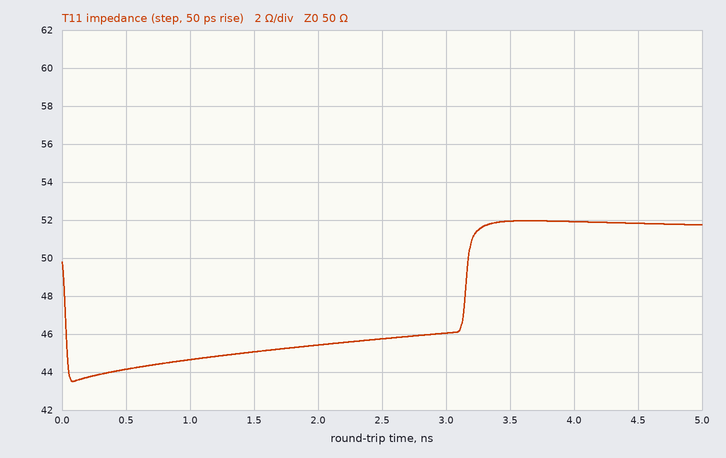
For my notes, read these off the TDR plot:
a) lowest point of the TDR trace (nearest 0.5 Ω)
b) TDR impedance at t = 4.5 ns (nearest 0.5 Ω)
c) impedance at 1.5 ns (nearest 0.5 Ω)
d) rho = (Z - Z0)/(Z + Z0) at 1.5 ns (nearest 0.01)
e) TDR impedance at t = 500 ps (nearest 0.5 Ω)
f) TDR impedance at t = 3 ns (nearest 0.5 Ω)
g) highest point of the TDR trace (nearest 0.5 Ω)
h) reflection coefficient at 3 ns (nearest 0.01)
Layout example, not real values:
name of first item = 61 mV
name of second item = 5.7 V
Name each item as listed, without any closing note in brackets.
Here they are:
lowest point of the TDR trace = 43.5 Ω
TDR impedance at t = 4.5 ns = 52.0 Ω
impedance at 1.5 ns = 45.0 Ω
rho = (Z - Z0)/(Z + Z0) at 1.5 ns = -0.05
TDR impedance at t = 500 ps = 44.0 Ω
TDR impedance at t = 3 ns = 46.0 Ω
highest point of the TDR trace = 52.0 Ω
reflection coefficient at 3 ns = -0.04
